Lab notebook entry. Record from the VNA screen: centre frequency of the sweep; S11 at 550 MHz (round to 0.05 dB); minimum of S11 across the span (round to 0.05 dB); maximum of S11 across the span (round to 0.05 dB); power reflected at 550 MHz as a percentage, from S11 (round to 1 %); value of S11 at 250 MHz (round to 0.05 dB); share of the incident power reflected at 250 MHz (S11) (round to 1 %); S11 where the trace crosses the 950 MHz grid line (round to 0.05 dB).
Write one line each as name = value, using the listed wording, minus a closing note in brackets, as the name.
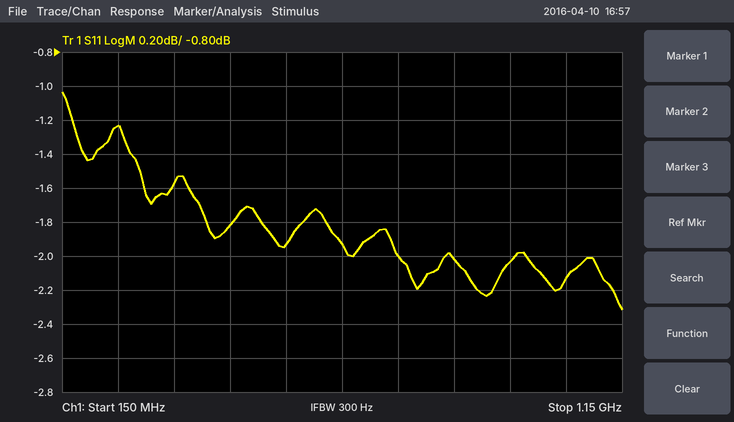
centre frequency of the sweep = 650 MHz
S11 at 550 MHz = -1.95 dB
minimum of S11 across the span = -2.30 dB
maximum of S11 across the span = -1.05 dB
power reflected at 550 MHz as a percentage, from S11 = 64 %
value of S11 at 250 MHz = -1.25 dB
share of the incident power reflected at 250 MHz (S11) = 75 %
S11 where the trace crosses the 950 MHz grid line = -2.05 dB
